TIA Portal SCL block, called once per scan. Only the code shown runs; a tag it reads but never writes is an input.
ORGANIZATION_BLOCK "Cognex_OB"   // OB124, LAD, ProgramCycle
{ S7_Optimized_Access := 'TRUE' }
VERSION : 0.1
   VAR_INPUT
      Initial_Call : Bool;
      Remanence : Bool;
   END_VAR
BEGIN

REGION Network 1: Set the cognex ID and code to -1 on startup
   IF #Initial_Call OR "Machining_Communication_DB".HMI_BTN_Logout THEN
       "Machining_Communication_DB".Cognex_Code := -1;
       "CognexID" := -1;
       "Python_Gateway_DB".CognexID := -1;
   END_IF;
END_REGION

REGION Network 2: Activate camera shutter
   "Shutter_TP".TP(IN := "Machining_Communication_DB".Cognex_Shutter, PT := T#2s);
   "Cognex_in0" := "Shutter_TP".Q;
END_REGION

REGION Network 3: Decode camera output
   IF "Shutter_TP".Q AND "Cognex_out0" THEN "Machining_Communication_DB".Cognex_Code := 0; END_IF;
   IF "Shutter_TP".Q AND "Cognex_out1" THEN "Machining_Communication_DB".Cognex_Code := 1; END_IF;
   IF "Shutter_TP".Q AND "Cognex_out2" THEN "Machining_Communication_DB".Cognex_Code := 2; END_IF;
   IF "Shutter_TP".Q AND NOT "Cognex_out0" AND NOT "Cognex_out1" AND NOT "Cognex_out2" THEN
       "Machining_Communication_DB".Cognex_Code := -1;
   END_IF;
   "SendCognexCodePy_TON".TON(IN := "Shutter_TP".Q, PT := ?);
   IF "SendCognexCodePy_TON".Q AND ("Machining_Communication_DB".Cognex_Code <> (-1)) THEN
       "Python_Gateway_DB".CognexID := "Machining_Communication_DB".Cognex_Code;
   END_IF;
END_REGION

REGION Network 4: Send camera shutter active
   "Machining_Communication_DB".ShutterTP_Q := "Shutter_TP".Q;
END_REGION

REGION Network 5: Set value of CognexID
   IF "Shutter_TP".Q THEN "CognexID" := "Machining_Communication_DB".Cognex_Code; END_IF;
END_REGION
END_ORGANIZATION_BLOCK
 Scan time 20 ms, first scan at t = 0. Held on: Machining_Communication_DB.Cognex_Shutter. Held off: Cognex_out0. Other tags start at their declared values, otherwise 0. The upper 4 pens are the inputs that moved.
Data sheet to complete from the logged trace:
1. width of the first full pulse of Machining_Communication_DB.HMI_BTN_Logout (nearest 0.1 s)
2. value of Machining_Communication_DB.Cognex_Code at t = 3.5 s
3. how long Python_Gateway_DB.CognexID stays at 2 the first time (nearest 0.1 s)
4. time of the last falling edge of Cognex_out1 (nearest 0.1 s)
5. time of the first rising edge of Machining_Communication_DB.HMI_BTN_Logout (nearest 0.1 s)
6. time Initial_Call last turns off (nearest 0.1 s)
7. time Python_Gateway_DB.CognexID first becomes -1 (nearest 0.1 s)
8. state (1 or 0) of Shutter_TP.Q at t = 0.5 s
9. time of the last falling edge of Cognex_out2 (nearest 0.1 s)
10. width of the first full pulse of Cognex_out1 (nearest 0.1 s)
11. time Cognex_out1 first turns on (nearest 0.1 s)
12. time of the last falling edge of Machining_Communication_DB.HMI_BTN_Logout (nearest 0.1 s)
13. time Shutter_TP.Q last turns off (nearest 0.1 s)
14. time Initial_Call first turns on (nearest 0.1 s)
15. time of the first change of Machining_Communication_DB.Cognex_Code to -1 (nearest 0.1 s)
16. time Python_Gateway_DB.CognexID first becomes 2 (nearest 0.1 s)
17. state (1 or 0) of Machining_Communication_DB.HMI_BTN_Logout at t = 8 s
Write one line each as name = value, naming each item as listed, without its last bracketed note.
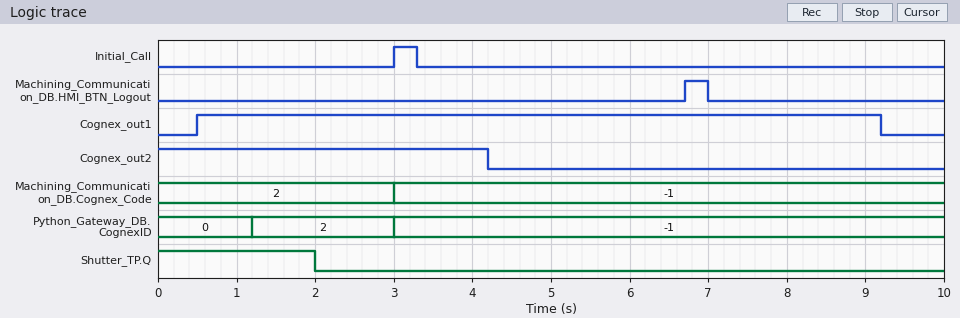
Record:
width of the first full pulse of Machining_Communication_DB.HMI_BTN_Logout = 0.3 s
value of Machining_Communication_DB.Cognex_Code at t = 3.5 s = -1
how long Python_Gateway_DB.CognexID stays at 2 the first time = 1.8 s
time of the last falling edge of Cognex_out1 = 9.2 s
time of the first rising edge of Machining_Communication_DB.HMI_BTN_Logout = 6.7 s
time Initial_Call last turns off = 3.3 s
time Python_Gateway_DB.CognexID first becomes -1 = 3.0 s
state (1 or 0) of Shutter_TP.Q at t = 0.5 s = 1
time of the last falling edge of Cognex_out2 = 4.2 s
width of the first full pulse of Cognex_out1 = 8.7 s
time Cognex_out1 first turns on = 0.5 s
time of the last falling edge of Machining_Communication_DB.HMI_BTN_Logout = 7.0 s
time Shutter_TP.Q last turns off = 2.0 s
time Initial_Call first turns on = 3.0 s
time of the first change of Machining_Communication_DB.Cognex_Code to -1 = 3.0 s
time Python_Gateway_DB.CognexID first becomes 2 = 1.2 s
state (1 or 0) of Machining_Communication_DB.HMI_BTN_Logout at t = 8 s = 0
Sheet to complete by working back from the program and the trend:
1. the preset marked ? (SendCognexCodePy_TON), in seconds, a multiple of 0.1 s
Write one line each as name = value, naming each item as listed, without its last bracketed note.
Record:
the preset marked ? (SendCognexCodePy_TON), in seconds, a multiple of 0.1 s = 1.2 s
